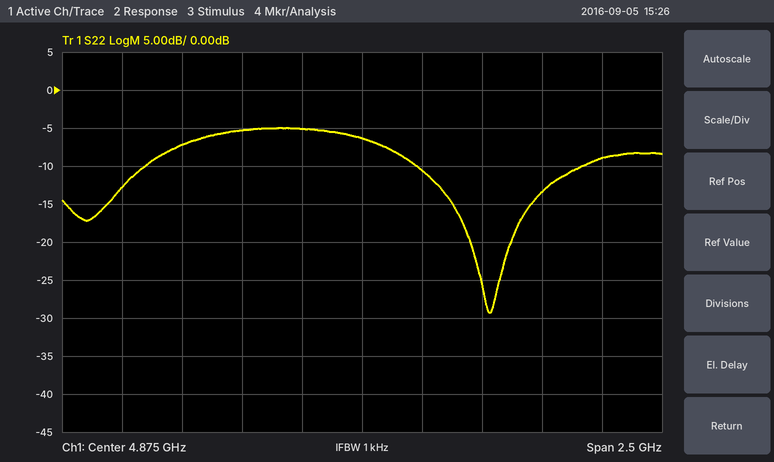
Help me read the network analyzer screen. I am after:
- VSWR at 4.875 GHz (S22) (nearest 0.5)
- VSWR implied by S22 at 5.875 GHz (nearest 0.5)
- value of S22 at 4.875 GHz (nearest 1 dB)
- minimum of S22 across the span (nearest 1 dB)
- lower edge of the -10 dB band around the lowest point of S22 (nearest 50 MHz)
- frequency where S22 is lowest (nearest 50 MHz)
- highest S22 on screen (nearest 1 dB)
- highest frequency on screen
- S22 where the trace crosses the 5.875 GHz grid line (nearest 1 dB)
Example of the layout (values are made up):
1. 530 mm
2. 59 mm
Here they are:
1. 3.0
2. 2.0
3. -6 dB
4. -29 dB
5. 5.10 GHz
6. 5.40 GHz
7. -5 dB
8. 6.125 GHz
9. -9 dB
